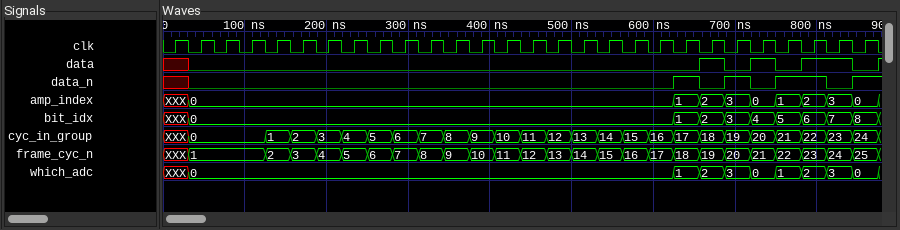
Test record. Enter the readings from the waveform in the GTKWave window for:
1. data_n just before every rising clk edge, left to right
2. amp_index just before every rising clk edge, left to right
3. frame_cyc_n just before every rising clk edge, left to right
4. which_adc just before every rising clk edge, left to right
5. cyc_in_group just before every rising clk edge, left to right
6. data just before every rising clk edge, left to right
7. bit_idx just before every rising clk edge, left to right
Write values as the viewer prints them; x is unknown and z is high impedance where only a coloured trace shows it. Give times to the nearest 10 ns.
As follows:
x 0 0 0 0 0 0 0 0 0 0 0 0 0 0 0 0 0 0 0 1 0 1 0 1 1 0 1
XXX, 0, 0, 0, 0, 0, 0, 0, 0, 0, 0, 0, 0, 0, 0, 0, 0, 0, 0, 0, 1, 2, 3, 0, 1, 2, 3, 0
XXX, 1, 1, 1, 2, 3, 4, 5, 6, 7, 8, 9, 10, 11, 12, 13, 14, 15, 16, 17, 18, 19, 20, 21, 22, 23, 24, 25
XXX, 0, 0, 0, 0, 0, 0, 0, 0, 0, 0, 0, 0, 0, 0, 0, 0, 0, 0, 0, 1, 2, 3, 0, 1, 2, 3, 0
XXX, 0, 0, 0, 1, 2, 3, 4, 5, 6, 7, 8, 9, 10, 11, 12, 13, 14, 15, 16, 17, 18, 19, 20, 21, 22, 23, 24
x 0 0 0 0 0 0 0 0 0 0 0 0 0 0 0 0 0 0 0 0 1 0 1 0 1 1 0
XXX, 0, 0, 0, 0, 0, 0, 0, 0, 0, 0, 0, 0, 0, 0, 0, 0, 0, 0, 0, 1, 2, 3, 4, 5, 6, 7, 8
